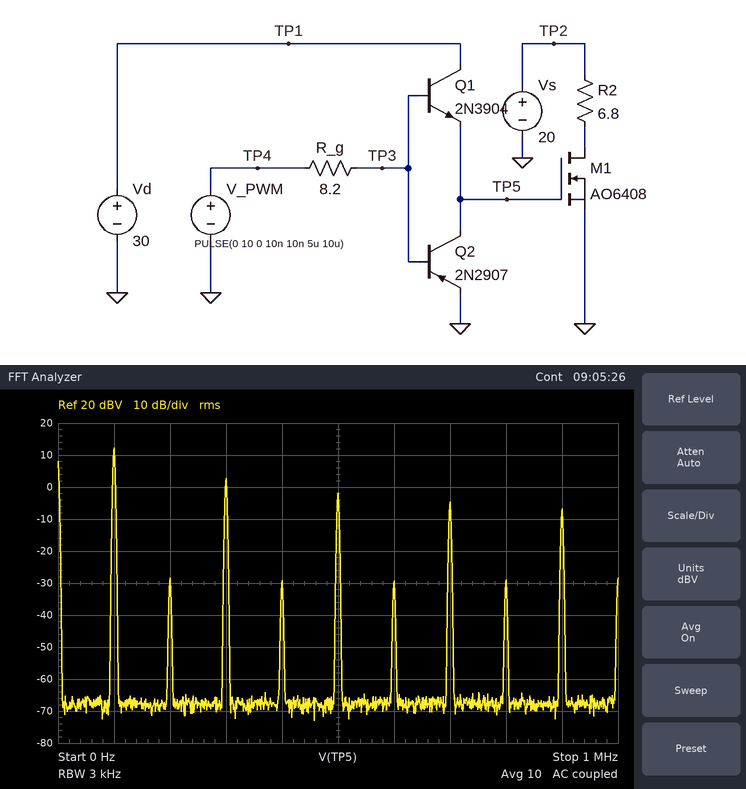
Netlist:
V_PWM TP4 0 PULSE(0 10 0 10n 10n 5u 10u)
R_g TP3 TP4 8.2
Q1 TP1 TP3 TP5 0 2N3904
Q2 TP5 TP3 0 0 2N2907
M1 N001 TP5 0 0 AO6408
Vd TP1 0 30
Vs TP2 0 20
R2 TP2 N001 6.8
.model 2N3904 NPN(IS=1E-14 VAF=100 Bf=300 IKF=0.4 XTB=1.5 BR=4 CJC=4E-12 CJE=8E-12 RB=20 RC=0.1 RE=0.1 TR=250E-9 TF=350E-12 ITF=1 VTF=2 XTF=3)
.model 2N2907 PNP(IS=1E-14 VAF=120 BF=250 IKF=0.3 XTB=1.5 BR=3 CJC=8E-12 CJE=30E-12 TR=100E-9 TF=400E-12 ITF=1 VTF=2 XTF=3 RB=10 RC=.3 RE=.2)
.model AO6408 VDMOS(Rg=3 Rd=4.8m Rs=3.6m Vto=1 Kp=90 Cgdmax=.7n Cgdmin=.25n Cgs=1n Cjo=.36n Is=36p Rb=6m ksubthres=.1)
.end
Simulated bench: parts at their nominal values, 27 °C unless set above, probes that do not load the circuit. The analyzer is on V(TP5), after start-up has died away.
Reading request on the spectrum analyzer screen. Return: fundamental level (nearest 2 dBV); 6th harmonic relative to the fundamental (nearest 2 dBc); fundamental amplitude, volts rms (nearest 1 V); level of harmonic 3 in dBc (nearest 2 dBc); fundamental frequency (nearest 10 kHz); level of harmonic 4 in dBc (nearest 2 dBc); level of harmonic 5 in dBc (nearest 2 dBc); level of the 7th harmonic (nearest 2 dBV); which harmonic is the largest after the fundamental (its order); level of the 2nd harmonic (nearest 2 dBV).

12 dBV
-42 dBc
4 V
-10 dBc
100 kHz
-42 dBc
-14 dBc
-4 dBV
3
-28 dBV
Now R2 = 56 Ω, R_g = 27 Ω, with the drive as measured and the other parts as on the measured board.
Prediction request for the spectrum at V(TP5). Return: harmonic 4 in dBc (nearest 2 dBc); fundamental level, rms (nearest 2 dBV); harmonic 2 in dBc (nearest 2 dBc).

-38 dBc
12 dBV
-38 dBc
